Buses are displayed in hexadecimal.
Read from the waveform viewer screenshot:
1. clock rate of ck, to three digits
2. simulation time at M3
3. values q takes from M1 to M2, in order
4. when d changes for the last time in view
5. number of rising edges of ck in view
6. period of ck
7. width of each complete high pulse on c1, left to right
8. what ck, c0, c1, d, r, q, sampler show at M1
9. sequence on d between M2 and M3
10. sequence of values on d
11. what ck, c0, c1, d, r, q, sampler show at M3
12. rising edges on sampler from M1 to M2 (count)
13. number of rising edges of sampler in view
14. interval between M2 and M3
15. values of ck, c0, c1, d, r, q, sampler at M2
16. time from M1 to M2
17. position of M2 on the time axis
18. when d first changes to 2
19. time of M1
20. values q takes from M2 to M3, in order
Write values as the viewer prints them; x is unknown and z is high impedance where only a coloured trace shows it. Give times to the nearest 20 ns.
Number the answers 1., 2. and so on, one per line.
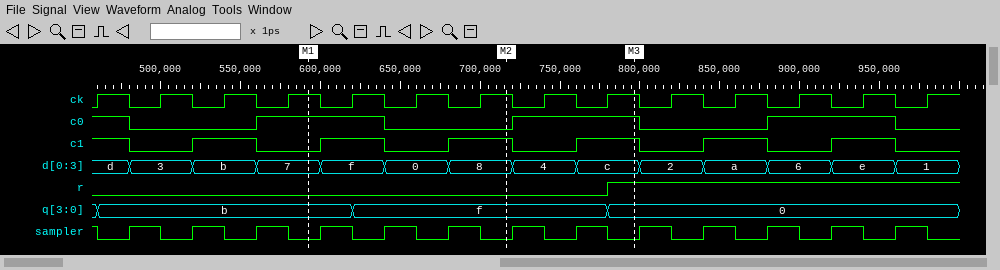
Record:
1. 25.0 MHz
2. 800 ns
3. b, f
4. 960 ns
5. 14
6. 40 ns
7. 40 ns, 40 ns, 40 ns, 40 ns, 40 ns, 40 ns
8. ck=1, c0=1, c1=0, d=7, r=0, q=b, sampler=0
9. 8, 4, c
10. d, 3, b, 7, f, 0, 8, 4, c, 2, a, 6, e, 1
11. ck=1, c0=1, c1=1, d=c, r=1, q=0, sampler=0
12. 3
13. 13
14. 80 ns
15. ck=1, c0=0, c1=1, d=8, r=0, q=f, sampler=0
16. 120 ns
17. 720 ns
18. 800 ns
19. 600 ns
20. f, 0
